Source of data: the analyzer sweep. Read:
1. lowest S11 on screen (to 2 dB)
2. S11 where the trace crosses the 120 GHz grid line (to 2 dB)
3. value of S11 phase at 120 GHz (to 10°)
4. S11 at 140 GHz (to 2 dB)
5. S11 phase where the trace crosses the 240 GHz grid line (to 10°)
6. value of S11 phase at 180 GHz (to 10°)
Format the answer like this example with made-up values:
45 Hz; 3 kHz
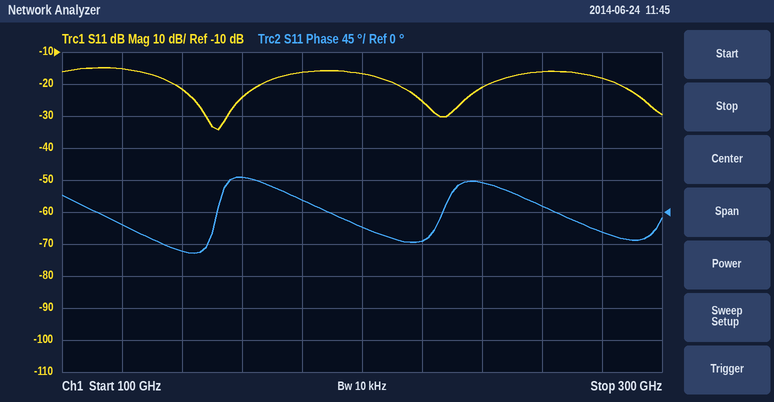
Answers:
-34 dB; -16 dB; -20°; -22 dB; 40°; 20°
